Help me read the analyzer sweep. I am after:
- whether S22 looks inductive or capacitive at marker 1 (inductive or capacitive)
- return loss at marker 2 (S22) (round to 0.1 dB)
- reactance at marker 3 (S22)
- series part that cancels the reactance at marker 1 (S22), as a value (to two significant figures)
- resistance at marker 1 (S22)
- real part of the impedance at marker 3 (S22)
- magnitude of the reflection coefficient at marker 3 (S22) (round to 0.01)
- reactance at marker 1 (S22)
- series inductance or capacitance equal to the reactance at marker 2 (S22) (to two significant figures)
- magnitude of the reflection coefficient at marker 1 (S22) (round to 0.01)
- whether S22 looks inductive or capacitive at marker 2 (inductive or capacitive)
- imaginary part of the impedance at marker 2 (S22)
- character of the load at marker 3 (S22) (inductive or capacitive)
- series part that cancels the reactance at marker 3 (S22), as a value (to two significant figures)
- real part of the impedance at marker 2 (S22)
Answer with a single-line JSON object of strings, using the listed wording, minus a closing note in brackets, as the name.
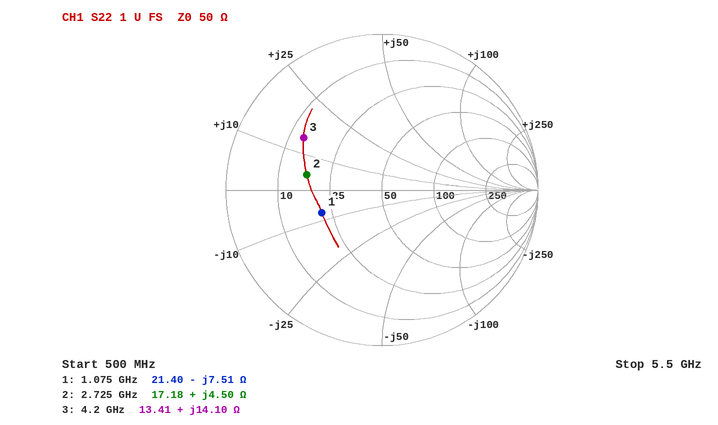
{"whether S22 looks inductive or capacitive at marker 1": "capacitive", "return loss at marker 2 (S22)": "6.2 dB", "reactance at marker 3": "+14.10 Ω", "series part that cancels the reactance at marker 1 (S22), as a value": "1.1 nH", "resistance at marker 1": "21.40 Ω", "real part of the impedance at marker 3": "13.41 Ω", "magnitude of the reflection coefficient at marker 3 (S22)": "0.60", "reactance at marker 1": "-7.51 Ω", "series inductance or capacitance equal to the reactance at marker 2 (S22)": "260 pH", "magnitude of the reflection coefficient at marker 1 (S22)": "0.41", "whether S22 looks inductive or capacitive at marker 2": "inductive", "imaginary part of the impedance at marker 2": "+4.50 Ω", "character of the load at marker 3 (S22)": "inductive", "series part that cancels the reactance at marker 3 (S22), as a value": "2.7 pF", "real part of the impedance at marker 2": "17.18 Ω"}
